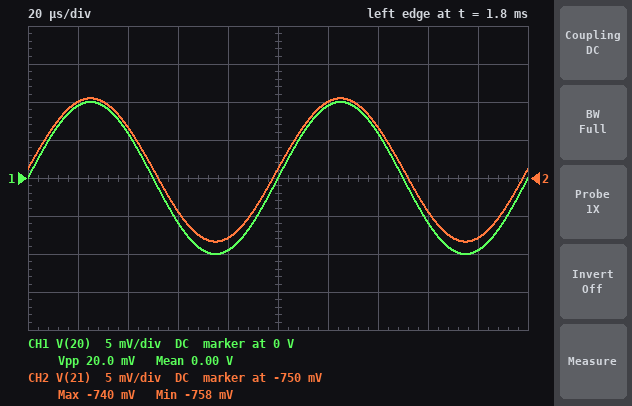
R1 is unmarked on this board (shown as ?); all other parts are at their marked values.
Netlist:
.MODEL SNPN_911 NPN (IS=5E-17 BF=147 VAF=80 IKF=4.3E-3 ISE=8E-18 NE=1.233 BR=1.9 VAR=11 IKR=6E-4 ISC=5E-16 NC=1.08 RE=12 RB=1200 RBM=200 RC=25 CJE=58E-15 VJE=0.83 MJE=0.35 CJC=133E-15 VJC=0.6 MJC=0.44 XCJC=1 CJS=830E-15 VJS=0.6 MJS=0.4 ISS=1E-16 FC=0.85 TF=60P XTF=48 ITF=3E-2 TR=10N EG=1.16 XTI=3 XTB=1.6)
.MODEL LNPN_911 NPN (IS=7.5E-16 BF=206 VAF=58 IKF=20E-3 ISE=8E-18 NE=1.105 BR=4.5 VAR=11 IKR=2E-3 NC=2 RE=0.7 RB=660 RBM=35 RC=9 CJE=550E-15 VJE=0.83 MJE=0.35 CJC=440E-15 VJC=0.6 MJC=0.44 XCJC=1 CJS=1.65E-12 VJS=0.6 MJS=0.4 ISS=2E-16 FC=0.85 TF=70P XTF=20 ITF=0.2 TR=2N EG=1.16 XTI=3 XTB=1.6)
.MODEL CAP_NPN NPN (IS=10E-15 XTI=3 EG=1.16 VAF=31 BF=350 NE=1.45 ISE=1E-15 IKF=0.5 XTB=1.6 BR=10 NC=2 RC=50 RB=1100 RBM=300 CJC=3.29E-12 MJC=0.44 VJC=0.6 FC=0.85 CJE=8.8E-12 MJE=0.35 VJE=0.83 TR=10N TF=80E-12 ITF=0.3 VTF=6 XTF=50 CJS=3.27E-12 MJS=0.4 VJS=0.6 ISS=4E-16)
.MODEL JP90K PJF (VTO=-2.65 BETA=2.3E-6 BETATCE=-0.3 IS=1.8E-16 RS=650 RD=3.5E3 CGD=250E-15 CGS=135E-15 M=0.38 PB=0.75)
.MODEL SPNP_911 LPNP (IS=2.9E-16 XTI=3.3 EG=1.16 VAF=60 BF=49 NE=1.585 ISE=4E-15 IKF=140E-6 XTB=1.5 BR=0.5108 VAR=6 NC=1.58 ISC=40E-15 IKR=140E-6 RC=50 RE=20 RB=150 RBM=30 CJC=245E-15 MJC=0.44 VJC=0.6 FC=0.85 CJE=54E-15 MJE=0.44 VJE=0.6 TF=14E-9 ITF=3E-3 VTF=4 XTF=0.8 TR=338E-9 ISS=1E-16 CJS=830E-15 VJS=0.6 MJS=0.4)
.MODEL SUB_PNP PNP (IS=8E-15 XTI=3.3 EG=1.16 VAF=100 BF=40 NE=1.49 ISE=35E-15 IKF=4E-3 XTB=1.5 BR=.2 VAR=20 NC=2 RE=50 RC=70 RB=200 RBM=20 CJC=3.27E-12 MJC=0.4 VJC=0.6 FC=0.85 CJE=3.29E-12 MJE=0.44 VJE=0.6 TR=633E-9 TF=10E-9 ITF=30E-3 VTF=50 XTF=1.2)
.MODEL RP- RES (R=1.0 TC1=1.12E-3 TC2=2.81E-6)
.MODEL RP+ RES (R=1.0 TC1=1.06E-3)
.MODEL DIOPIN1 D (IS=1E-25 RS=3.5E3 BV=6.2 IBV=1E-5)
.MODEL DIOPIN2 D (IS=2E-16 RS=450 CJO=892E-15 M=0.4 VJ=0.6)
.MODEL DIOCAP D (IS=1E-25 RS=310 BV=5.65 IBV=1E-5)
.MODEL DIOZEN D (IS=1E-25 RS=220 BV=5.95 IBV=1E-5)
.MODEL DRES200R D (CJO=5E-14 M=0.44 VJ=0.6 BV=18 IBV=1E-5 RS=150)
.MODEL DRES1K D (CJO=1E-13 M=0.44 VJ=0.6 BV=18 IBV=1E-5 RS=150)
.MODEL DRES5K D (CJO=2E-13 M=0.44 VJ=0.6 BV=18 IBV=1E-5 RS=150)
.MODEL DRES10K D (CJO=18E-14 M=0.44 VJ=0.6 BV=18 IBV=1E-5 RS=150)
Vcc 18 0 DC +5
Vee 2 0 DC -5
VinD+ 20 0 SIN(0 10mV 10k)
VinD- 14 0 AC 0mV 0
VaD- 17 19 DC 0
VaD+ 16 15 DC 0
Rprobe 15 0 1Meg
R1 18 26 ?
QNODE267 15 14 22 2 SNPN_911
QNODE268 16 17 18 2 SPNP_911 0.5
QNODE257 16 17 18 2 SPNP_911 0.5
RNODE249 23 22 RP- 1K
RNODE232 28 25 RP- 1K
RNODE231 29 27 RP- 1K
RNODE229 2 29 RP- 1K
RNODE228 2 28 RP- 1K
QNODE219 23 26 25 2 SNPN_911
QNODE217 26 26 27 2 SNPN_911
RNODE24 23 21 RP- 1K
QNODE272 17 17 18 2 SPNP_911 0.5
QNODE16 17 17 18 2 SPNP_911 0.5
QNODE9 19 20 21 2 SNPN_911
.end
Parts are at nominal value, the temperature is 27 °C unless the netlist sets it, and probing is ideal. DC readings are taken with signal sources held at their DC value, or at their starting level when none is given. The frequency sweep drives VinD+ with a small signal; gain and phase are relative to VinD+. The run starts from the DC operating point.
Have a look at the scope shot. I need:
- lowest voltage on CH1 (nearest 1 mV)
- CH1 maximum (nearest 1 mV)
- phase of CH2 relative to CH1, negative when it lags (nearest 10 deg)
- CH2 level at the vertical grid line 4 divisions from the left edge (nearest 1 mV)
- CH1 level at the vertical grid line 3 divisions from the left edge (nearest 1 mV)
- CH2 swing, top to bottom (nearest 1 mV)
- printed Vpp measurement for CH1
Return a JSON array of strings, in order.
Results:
["-10 mV", "10 mV", "0 deg", "-758 mV", "-6 mV", "19 mV", "20.0 mV"]
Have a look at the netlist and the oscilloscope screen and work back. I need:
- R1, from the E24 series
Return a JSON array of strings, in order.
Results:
["27 kΩ"]
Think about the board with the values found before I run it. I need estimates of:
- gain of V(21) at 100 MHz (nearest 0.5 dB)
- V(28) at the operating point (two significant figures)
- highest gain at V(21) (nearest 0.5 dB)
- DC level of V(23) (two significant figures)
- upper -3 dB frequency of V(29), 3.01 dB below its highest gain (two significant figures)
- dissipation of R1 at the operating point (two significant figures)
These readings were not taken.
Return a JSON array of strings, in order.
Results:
["-0.5 dB", "-4.7 V", "-0.5 dB", "-910 mV", "540 MHz", "2.7 mW"]
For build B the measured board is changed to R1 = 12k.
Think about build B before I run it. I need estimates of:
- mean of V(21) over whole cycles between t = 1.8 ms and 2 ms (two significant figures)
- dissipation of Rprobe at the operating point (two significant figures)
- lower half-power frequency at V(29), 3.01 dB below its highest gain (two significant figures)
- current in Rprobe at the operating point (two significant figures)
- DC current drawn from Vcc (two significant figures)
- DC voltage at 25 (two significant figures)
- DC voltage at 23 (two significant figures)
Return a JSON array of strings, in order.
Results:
["-770 mV", "430 nW", "90 MHz", "660 nA", "1.3 mA", "-3.7 V", "-1.1 V"]
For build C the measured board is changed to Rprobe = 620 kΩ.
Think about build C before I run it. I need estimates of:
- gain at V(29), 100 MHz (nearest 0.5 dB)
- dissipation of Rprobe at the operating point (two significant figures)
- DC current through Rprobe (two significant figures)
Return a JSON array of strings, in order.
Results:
["-36.0 dB", "450 nW", "850 nA"]
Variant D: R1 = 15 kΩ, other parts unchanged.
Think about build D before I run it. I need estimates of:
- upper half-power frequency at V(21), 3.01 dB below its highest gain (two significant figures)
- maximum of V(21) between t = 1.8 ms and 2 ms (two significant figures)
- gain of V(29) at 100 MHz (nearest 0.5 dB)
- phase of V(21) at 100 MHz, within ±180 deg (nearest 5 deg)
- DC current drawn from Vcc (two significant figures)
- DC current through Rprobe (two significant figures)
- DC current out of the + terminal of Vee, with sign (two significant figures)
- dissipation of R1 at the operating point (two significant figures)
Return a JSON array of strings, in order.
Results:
["1.0 GHz", "-760 mV", "-34.5 dB", "-5 deg", "1.1 mA", "640 nA", "-1.1 mA", "4.4 mW"]
